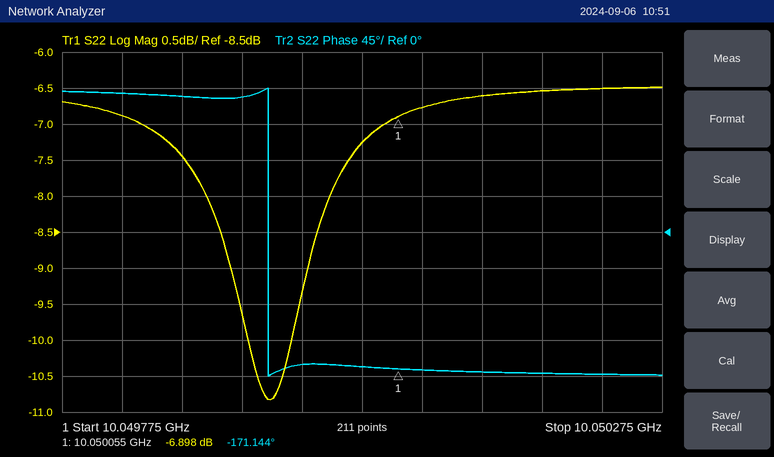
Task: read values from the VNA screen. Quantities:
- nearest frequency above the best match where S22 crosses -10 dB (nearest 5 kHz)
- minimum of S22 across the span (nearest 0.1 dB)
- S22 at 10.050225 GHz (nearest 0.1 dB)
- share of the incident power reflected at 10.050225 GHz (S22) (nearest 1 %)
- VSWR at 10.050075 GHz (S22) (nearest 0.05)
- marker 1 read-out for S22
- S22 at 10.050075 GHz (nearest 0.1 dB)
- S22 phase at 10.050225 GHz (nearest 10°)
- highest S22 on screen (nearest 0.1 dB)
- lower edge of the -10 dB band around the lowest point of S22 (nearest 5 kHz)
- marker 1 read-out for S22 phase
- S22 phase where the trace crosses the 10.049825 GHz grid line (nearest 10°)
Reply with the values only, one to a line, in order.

10.049965 GHz
-10.8 dB
-6.5 dB
22 %
2.70
-6.898 dB
-6.8 dB
-180°
-6.5 dB
10.049930 GHz
-171.144°
170°
